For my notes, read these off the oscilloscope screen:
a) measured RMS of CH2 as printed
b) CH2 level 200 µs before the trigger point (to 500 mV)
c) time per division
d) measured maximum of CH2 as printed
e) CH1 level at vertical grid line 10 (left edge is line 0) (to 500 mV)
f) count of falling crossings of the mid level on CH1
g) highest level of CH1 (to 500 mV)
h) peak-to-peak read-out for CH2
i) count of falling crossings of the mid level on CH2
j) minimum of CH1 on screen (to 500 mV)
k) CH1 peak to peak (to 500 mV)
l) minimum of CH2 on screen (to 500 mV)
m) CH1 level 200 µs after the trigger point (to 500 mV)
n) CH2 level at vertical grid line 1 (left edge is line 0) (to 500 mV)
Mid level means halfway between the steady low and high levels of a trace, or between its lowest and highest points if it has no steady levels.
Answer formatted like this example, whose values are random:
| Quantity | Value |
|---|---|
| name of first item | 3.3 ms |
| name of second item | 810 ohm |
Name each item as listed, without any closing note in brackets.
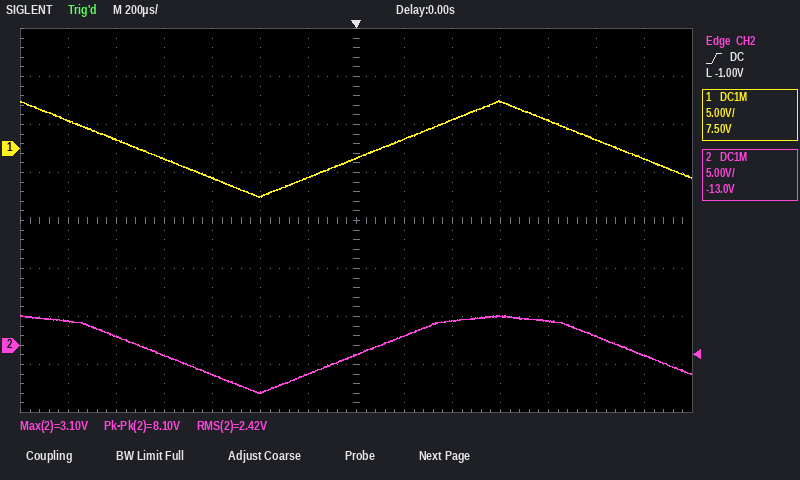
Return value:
| Quantity | Value |
|---|---|
| measured RMS of CH2 as printed | 2.42 V |
| CH2 level 200 µs before the trigger point | -3.0 V |
| time per division | 200 µs |
| measured maximum of CH2 as printed | 3.10 V |
| CH1 level at vertical grid line 10 (left edge is line 0) | 5.0 V |
| count of falling crossings of the mid level on CH1 | 2 |
| highest level of CH1 | 5.0 V |
| peak-to-peak read-out for CH2 | 8.10 V |
| count of falling crossings of the mid level on CH2 | 2 |
| minimum of CH1 on screen | -5.0 V |
| CH1 peak to peak | 10.0 V |
| minimum of CH2 on screen | -5.0 V |
| CH1 level 200 µs after the trigger point | 1.0 V |
| CH2 level at vertical grid line 1 (left edge is line 0) | 2.5 V |
